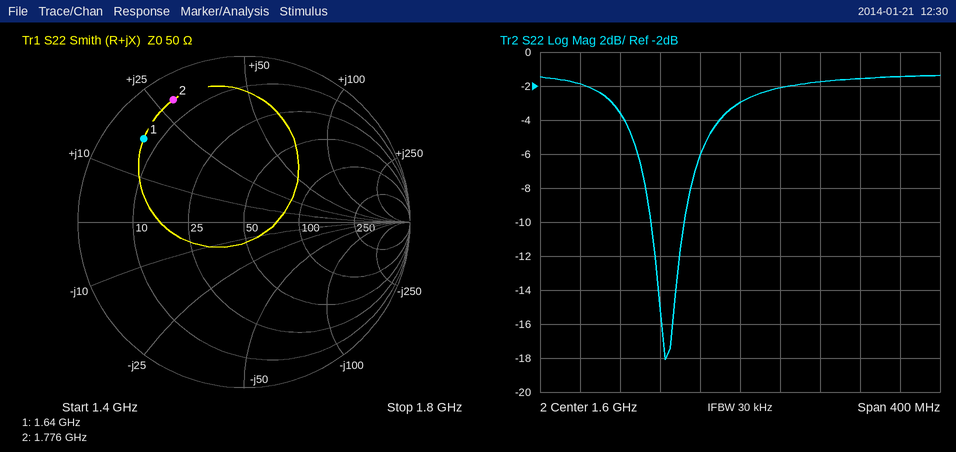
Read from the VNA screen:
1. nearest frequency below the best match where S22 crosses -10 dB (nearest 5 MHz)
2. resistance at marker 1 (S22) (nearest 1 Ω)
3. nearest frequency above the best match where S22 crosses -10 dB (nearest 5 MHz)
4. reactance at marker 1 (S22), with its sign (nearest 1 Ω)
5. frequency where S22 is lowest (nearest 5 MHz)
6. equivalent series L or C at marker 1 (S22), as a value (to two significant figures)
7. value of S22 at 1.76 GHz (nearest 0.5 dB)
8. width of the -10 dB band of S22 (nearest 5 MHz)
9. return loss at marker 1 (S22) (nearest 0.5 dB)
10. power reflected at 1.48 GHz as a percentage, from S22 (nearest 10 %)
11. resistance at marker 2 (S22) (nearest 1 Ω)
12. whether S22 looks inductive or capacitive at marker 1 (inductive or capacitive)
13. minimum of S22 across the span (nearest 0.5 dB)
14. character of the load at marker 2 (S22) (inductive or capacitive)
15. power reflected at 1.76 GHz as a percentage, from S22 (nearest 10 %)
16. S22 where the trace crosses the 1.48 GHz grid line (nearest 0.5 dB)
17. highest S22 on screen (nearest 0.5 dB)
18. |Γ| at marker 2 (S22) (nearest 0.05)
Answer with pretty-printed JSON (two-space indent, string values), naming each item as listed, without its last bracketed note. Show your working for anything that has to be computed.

{
  "nearest frequency below the best match where S22 crosses -10 dB": "1.510 GHz",
  "resistance at marker 1 (S22)": "7 Ω",
  "nearest frequency above the best match where S22 crosses -10 dB": "1.545 GHz",
  "reactance at marker 1 (S22), with its sign": "+18 Ω",
  "frequency where S22 is lowest": "1.525 GHz",
  "equivalent series L or C at marker 1 (S22), as a value": "L = 18 Ω/(2π × 1.64 GHz) ≈ 1.7 nH",
  "value of S22 at 1.76 GHz": "-1.5 dB",
  "width of the -10 dB band of S22": "1.545 GHz − 1.510 GHz = 35 MHz",
  "return loss at marker 1 (S22)": "2.0 dB",
  "power reflected at 1.48 GHz as a percentage, from S22": "10^(-3.5/10) ≈ 44.7 %, so 40 % to the nearest 10 %",
  "resistance at marker 2 (S22)": "5 Ω",
  "whether S22 looks inductive or capacitive at marker 1": "inductive",
  "minimum of S22 across the span": "-18.0 dB",
  "character of the load at marker 2 (S22)": "inductive",
  "power reflected at 1.76 GHz as a percentage, from S22": "10^(-1.5/10) ≈ 70.8 %, so 70 % to the nearest 10 %",
  "S22 where the trace crosses the 1.48 GHz grid line": "-3.5 dB",
  "highest S22 on screen": "-1.5 dB",
  "|Γ| at marker 2 (S22)": "0.85"
}
